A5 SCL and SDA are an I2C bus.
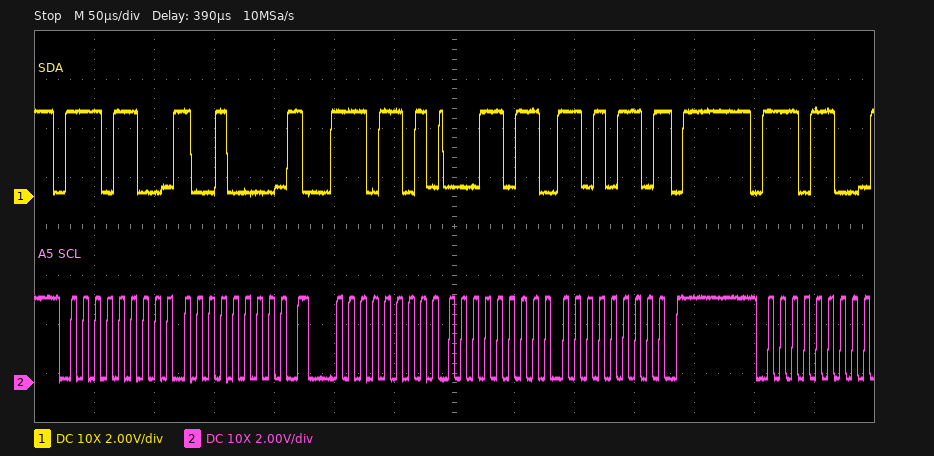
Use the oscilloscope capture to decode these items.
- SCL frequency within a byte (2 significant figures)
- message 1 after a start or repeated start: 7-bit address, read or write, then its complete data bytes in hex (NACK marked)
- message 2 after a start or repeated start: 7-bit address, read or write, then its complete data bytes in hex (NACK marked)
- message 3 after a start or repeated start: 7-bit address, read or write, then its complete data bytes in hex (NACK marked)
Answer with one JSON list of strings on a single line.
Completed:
["100 kHz", "0x76 write: 90", "0x76 read: 1B D6 NACK", "0x76 write"]
